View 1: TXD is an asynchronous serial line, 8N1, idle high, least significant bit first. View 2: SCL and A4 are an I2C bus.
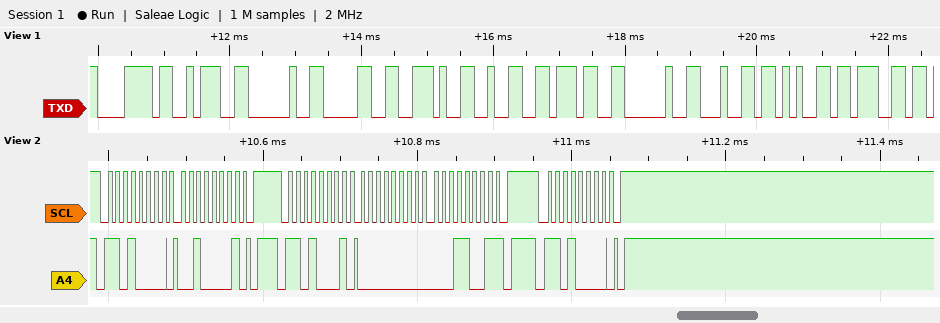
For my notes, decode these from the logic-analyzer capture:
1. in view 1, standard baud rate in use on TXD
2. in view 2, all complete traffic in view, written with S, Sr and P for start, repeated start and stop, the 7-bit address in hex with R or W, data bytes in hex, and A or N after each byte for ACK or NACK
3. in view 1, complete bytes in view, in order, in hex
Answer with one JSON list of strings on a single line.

["9600 baud", "S 68W A 21 A P S 68R A 00 A 19 N P S 68W A P", "0x78 0x3A 0x20 0x30 0x2E 0x32 0x37 0x20 0x64 0x65 0x67"]
